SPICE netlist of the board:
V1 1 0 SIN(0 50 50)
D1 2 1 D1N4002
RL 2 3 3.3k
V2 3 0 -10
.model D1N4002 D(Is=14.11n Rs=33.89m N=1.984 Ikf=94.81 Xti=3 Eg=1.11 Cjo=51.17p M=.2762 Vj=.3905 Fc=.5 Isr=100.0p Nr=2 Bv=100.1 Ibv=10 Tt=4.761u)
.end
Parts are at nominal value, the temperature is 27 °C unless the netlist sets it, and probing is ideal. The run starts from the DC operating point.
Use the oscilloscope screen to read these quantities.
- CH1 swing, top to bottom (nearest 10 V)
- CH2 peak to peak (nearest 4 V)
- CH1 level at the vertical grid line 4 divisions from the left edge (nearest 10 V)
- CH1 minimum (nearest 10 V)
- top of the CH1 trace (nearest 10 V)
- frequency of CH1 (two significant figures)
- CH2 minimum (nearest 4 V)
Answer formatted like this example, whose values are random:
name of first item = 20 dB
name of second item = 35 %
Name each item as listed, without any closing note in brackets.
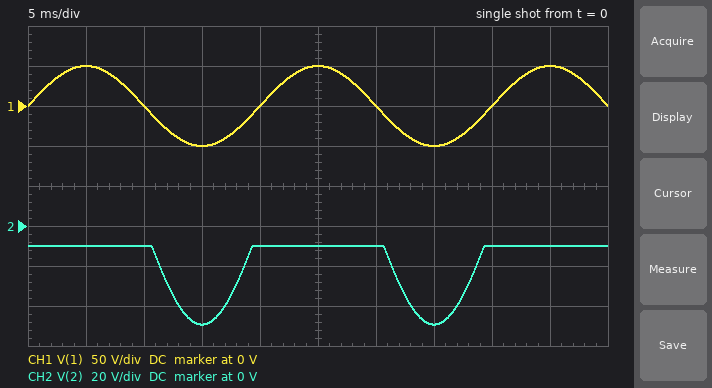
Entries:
CH1 swing, top to bottom = 100 V
CH2 peak to peak = 40 V
CH1 level at the vertical grid line 4 divisions from the left edge = 0 V
CH1 minimum = -50 V
top of the CH1 trace = 50 V
frequency of CH1 = 50 Hz
CH2 minimum = -48 V
